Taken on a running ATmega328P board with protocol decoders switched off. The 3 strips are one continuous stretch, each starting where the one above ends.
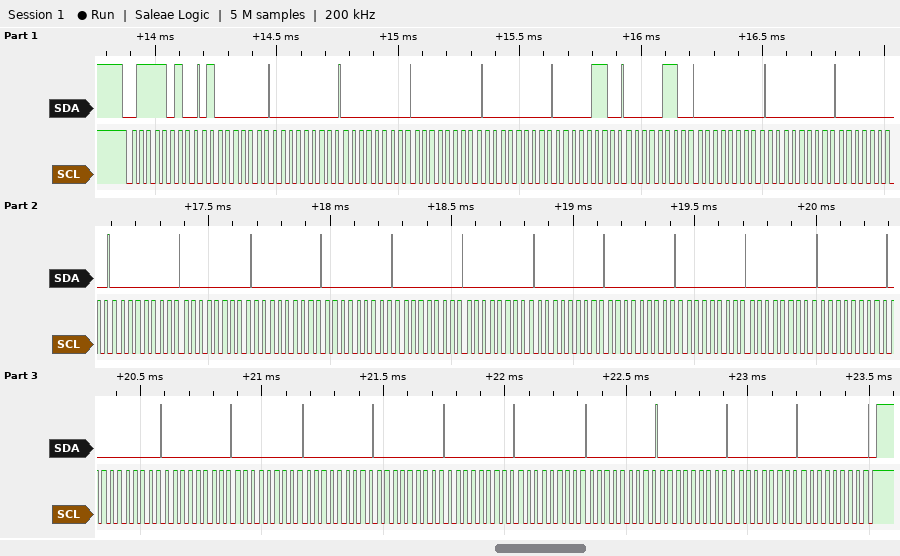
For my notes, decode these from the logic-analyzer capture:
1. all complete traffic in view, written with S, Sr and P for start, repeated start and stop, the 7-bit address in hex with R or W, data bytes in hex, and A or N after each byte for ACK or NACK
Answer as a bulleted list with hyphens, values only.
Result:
- S 3DW A 40 A 00 A 00 A 00 A 00 A 06 A 06 A 00 A 00 A 00 A 00 A 00 A 00 A 00 A 00 A 00 A 00 A 00 A 00 A 00 A 00 A 00 A 00 A 00 A 00 A 00 A 00 A 00 A 00 A 00 A 00 A 00 A P
